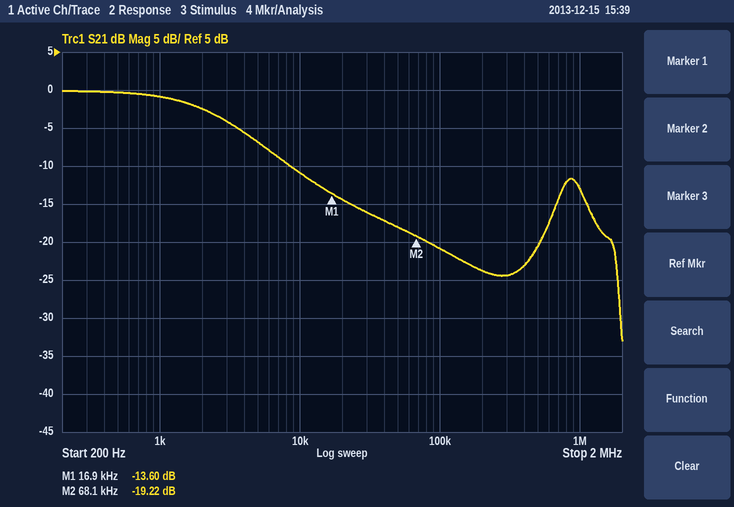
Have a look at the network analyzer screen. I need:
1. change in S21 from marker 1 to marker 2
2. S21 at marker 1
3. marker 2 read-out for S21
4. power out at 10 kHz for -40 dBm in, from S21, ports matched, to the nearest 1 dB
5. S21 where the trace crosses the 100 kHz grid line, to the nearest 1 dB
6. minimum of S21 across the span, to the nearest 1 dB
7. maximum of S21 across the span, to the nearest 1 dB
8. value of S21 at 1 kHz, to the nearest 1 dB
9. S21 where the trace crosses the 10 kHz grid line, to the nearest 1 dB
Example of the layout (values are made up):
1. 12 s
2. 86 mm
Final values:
1. -5.62 dB
2. -13.60 dB
3. -19.22 dB
4. -51 dBm
5. -21 dB
6. -33 dB
7. 0 dB
8. -1 dB
9. -11 dB
